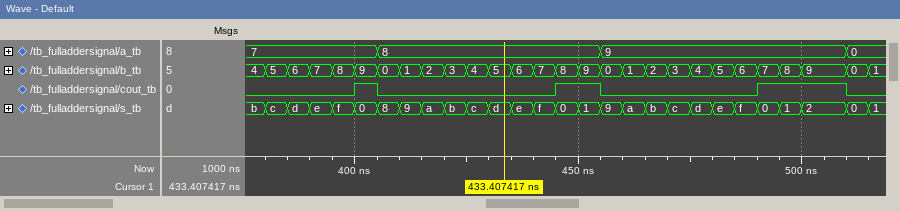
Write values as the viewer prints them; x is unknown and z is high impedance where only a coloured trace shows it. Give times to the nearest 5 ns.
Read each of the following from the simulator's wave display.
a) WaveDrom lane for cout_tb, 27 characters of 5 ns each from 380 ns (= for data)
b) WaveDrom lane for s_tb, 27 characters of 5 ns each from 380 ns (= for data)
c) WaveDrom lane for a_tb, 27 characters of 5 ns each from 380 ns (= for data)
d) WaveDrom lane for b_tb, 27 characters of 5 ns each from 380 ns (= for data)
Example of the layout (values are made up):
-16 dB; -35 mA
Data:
{name: 'cout_tb', wave: '0...10.......1.0......1...0'}; {name: 's_tb', wave: '=========================.=', data: 'c d e f 0 8 9 a b c d e f 0 1 9 a b c d e f 0 1 2 0'}; {name: 'a_tb', wave: '=....=.........=..........=', data: '7 8 9 0'}; {name: 'b_tb', wave: '=========================.=', data: '5 6 7 8 9 0 1 2 3 4 5 6 7 8 9 0 1 2 3 4 5 6 7 8 9 0'}
